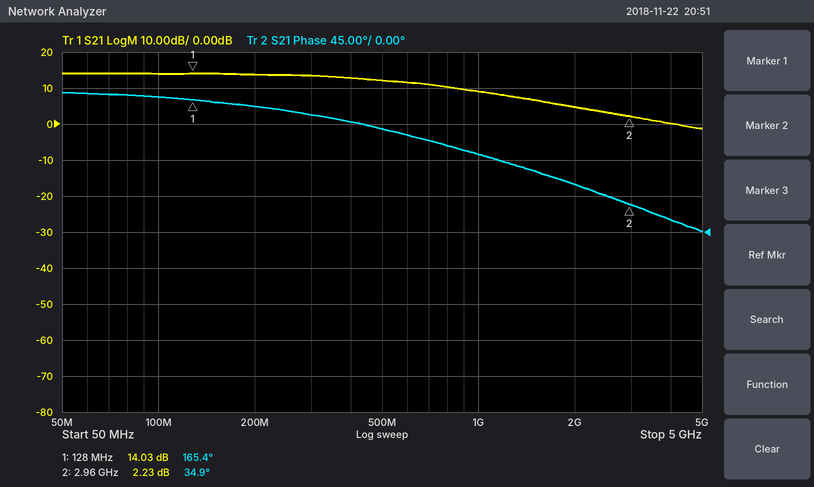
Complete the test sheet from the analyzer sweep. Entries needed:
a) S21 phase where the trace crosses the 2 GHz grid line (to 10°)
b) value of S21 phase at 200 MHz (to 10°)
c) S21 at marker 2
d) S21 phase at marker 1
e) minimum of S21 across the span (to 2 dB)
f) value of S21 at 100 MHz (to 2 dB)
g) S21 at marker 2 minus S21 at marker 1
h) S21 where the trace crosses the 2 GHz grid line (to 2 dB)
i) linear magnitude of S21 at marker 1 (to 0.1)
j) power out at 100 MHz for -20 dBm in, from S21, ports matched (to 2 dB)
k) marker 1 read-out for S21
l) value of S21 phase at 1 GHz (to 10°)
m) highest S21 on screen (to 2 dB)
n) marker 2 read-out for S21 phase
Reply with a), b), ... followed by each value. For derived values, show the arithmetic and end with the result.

a) 60°
b) 160°
c) 2.23 dB
d) 165.4°
e) -2 dB
f) 14 dB
g) 2.23 − (14.03) = -11.80 dB
h) 4 dB
i) 10^(14.03/20) ≈ 5.0
j) -20 dBm + (14 dB) = -6 dBm
k) 14.03 dB
l) 100°
m) 14 dB
n) 34.9°
